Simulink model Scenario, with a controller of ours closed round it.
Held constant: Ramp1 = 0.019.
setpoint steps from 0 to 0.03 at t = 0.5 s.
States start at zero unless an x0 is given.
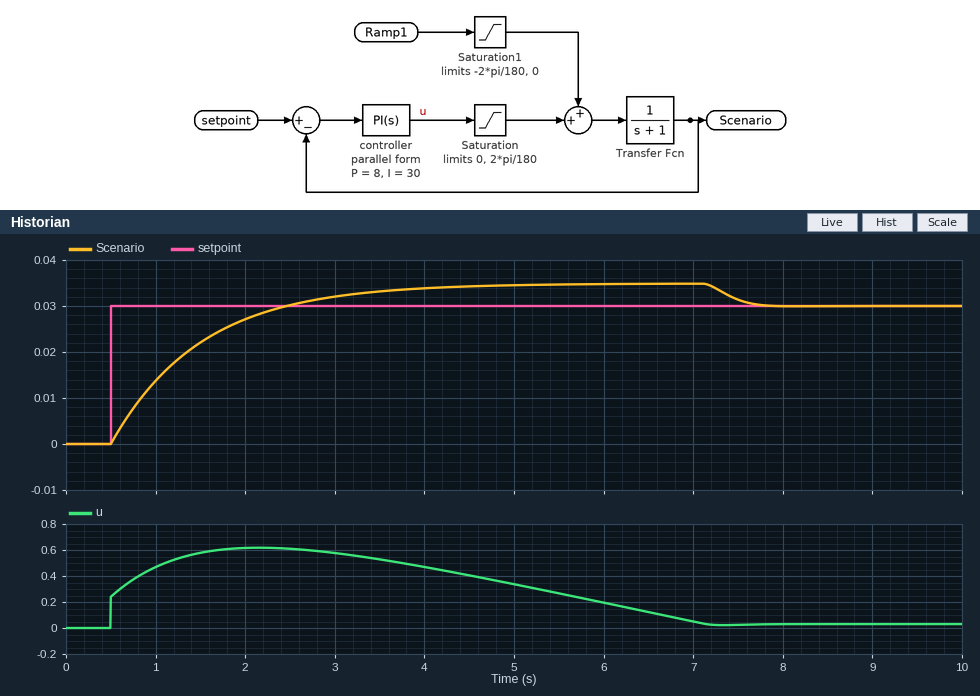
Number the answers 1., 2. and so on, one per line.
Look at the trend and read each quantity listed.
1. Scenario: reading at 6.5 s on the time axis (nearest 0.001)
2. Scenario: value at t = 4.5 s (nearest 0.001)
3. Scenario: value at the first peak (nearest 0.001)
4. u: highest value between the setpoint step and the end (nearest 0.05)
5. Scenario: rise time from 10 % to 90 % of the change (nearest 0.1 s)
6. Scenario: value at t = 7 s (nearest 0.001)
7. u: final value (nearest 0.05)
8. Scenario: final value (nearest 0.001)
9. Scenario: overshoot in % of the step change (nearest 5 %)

1. 0.035
2. 0.034
3. 0.035
4. 0.60
5. 1.4 s
6. 0.035
7. 0.05
8. 0.030
9. 15 %
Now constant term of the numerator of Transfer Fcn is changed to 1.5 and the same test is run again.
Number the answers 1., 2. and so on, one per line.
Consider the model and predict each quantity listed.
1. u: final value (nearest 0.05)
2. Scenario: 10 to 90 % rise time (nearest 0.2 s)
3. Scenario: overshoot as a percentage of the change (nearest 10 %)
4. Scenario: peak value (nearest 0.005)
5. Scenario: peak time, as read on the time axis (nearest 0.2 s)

1. 0.00
2. 0.6 s
3. 40 %
4. 0.045
5. 2.2 s
